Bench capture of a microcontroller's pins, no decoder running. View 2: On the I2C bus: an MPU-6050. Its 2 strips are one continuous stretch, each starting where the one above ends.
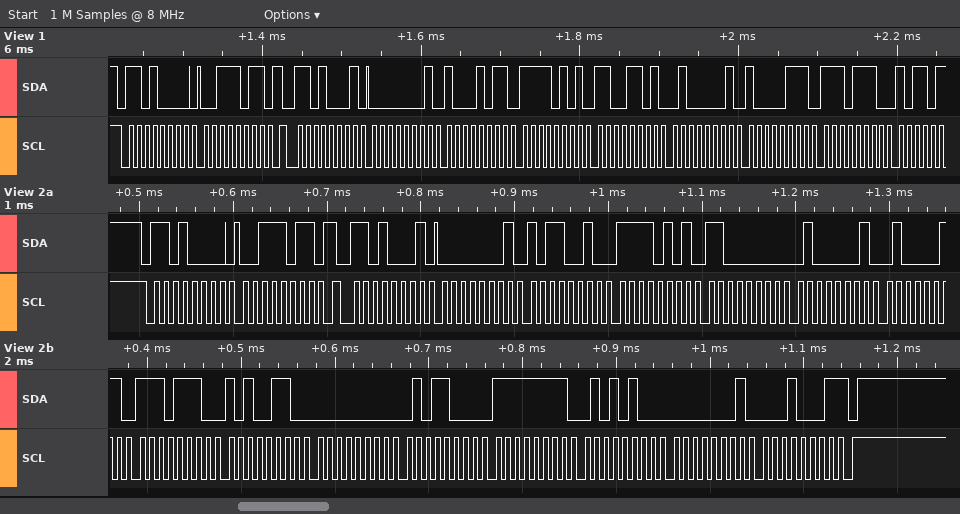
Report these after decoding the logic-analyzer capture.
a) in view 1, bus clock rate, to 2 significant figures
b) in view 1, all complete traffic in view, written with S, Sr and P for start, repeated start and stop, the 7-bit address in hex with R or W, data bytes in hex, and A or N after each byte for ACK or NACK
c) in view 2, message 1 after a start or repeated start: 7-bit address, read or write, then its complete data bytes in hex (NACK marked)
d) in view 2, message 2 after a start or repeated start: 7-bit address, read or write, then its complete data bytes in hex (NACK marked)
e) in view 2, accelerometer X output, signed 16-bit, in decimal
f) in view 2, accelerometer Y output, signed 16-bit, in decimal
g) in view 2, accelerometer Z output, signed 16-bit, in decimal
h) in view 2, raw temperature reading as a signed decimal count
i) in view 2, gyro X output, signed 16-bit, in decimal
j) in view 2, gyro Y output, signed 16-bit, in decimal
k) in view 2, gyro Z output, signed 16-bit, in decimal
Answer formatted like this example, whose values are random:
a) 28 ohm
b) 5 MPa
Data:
a) 100 kHz
b) S 68W A 3B A Sr 68R A 01 A 8B A F5 A CD A 41 A 87 A EE A
c) 0x68 write: 3B
d) 0x68 read: 01 B2 F5 C0 41 43 EE A6 00 58 FF 54 01 11 NACK
e) 434
f) -2624
g) 16707
h) -4442
i) 88
j) -172
k) 273
